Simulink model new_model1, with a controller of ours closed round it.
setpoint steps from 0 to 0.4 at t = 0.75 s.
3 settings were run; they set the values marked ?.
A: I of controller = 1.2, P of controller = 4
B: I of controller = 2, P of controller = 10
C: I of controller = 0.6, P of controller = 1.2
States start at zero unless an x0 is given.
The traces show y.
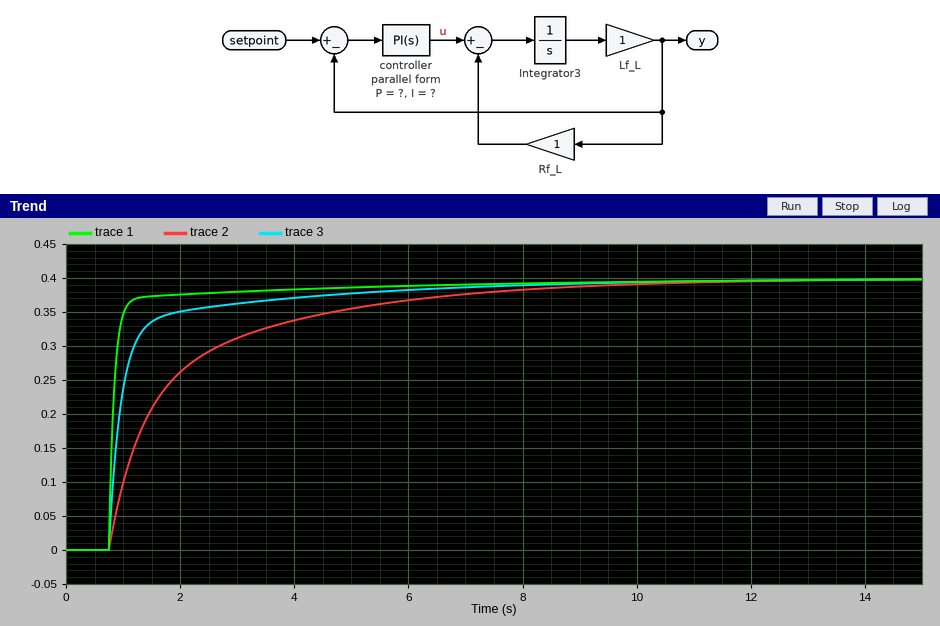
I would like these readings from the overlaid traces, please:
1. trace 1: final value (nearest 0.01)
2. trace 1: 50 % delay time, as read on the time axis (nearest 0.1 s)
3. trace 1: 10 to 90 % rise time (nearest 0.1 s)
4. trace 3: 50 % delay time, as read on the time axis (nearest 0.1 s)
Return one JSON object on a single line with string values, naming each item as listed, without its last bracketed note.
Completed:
{"trace 1: final value": "0.40", "trace 1: 50 % delay time, as read on the time axis": "0.8 s", "trace 1: 10 to 90 % rise time": "0.3 s", "trace 3: 50 % delay time, as read on the time axis": "0.9 s"}
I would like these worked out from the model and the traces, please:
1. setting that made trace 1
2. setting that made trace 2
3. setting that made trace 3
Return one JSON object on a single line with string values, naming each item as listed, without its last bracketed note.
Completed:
{"setting that made trace 1": "B", "setting that made trace 2": "C", "setting that made trace 3": "A"}
